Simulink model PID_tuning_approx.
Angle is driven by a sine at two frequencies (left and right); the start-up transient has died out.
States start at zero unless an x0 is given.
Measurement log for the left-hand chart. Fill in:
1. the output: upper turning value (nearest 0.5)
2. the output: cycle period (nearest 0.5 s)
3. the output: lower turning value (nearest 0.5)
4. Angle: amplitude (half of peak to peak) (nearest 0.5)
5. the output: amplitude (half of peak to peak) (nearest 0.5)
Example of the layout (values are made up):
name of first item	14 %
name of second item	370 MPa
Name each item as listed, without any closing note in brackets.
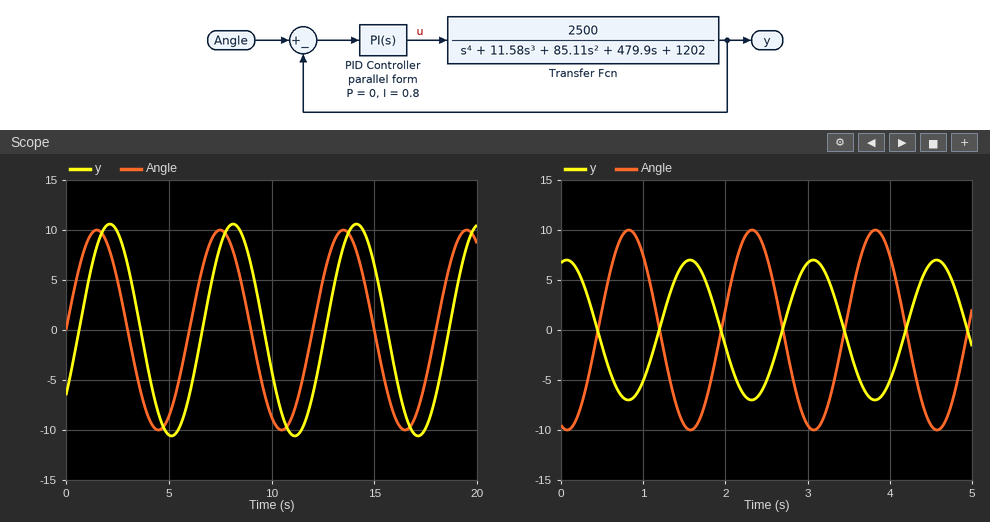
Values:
the output: upper turning value	10.5
the output: cycle period	6.0 s
the output: lower turning value	-10.5
Angle: amplitude (half of peak to peak)	10.0
the output: amplitude (half of peak to peak)	10.5
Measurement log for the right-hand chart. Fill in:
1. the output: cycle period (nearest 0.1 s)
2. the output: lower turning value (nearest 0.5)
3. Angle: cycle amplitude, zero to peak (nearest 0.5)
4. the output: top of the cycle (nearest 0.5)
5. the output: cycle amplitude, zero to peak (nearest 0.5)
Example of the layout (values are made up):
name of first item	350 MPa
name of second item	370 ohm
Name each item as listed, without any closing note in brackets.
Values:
the output: cycle period	1.5 s
the output: lower turning value	-7.0
Angle: cycle amplitude, zero to peak	10.0
the output: top of the cycle	7.0
the output: cycle amplitude, zero to peak	7.0
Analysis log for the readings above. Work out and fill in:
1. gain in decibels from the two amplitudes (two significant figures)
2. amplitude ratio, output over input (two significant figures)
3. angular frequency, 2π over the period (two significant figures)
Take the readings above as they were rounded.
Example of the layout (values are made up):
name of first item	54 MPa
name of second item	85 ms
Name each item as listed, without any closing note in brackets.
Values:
gain in decibels from the two amplitudes	-3.1 dB
amplitude ratio, output over input	0.70
angular frequency, 2π over the period	4.2 rad/s
